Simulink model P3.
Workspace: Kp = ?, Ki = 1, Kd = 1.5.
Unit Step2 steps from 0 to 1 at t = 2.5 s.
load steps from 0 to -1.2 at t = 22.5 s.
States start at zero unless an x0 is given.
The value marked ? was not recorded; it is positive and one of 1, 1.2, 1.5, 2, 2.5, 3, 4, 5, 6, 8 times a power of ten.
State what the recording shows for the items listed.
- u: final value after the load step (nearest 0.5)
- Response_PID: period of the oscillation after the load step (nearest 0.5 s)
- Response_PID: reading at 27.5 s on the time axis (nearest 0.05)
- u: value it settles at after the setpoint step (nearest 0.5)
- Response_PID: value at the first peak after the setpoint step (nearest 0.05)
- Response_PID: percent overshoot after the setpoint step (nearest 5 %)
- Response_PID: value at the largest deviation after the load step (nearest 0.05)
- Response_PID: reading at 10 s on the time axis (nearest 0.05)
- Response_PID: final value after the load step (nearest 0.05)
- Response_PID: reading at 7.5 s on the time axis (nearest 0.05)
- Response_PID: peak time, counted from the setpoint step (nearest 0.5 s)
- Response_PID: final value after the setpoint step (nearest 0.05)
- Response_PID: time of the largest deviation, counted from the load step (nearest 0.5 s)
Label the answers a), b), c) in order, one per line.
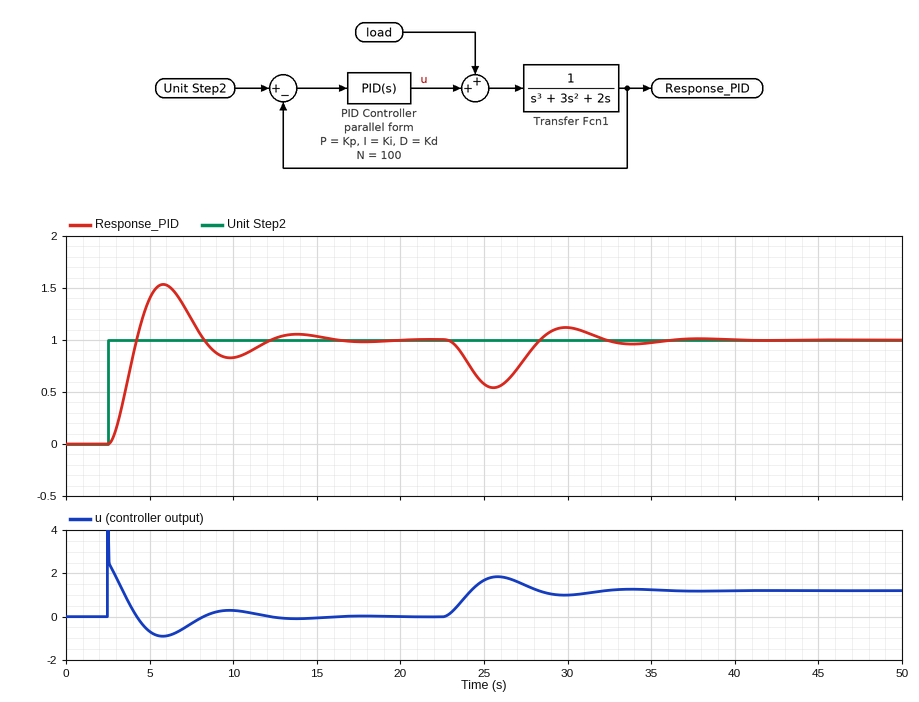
a) 1.0
b) 8.5 s
c) 0.85
d) 0.0
e) 1.55
f) 55 %
g) 0.55
h) 0.85
i) 1.00
j) 1.20
k) 3.5 s
l) 1.00
m) 3.0 s
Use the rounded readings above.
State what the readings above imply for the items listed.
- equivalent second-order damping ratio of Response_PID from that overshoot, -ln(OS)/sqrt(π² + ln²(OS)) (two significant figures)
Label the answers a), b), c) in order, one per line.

a) 0.19
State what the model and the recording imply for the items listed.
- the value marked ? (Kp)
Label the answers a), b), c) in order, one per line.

a) 2.5
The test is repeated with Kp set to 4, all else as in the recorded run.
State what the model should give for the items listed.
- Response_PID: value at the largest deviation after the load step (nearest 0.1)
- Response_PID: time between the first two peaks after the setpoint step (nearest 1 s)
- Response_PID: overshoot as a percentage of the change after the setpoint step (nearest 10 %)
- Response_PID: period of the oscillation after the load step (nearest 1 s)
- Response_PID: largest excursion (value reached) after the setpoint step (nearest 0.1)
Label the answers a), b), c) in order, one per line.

a) 0.6
b) 5 s
c) 60 %
d) 5 s
e) 1.6
